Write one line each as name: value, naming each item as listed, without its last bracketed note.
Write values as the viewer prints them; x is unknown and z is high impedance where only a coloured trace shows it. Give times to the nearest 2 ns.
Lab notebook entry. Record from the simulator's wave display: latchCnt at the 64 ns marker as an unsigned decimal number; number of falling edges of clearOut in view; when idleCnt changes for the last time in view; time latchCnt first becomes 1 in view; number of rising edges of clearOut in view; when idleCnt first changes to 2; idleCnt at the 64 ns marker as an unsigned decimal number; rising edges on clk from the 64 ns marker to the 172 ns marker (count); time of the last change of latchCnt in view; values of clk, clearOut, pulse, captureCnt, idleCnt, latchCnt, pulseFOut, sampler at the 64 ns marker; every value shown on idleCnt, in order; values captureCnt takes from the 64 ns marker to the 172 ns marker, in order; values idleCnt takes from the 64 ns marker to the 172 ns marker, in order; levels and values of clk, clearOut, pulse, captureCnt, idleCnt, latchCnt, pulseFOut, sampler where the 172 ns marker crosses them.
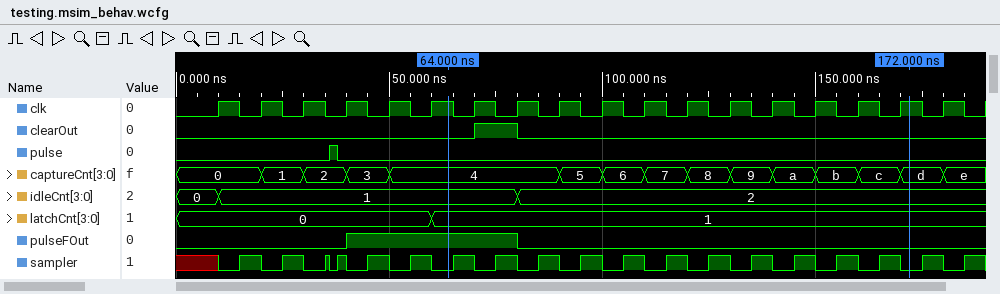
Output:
latchCnt at the 64 ns marker as an unsigned decimal number: 1
number of falling edges of clearOut in view: 1
when idleCnt changes for the last time in view: 80 ns
time latchCnt first becomes 1 in view: 60 ns
number of rising edges of clearOut in view: 1
when idleCnt first changes to 2: 80 ns
idleCnt at the 64 ns marker as an unsigned decimal number: 1
rising edges on clk from the 64 ns marker to the 172 ns marker: 11
time of the last change of latchCnt in view: 60 ns
values of clk, clearOut, pulse, captureCnt, idleCnt, latchCnt, pulseFOut, sampler at the 64 ns marker: clk=1, clearOut=0, pulse=0, captureCnt=4, idleCnt=1, latchCnt=1, pulseFOut=1, sampler=0
every value shown on idleCnt, in order: 0, 1, 2
values captureCnt takes from the 64 ns marker to the 172 ns marker, in order: 4, 5, 6, 7, 8, 9, a, b, c, d
values idleCnt takes from the 64 ns marker to the 172 ns marker, in order: 1, 2
levels and values of clk, clearOut, pulse, captureCnt, idleCnt, latchCnt, pulseFOut, sampler where the 172 ns marker crosses them: clk=1, clearOut=0, pulse=0, captureCnt=d, idleCnt=2, latchCnt=1, pulseFOut=0, sampler=0
